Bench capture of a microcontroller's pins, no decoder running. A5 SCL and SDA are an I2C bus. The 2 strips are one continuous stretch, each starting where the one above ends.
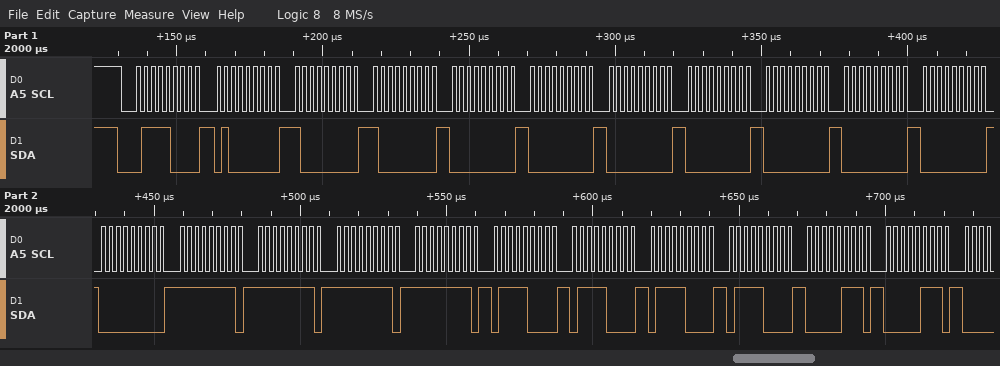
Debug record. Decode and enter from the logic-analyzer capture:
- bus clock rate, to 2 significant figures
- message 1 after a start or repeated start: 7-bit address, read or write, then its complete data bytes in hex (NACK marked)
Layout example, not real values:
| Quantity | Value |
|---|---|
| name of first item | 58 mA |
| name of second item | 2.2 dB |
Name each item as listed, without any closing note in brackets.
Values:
| Quantity | Value |
|---|---|
| bus clock rate, to 2 significant figures | 400 kHz |
| message 1 after a start or repeated start: 7-bit address, read or write, then its complete data bytes in hex | 0x3C write: 40 80 80 00 00 00 00 00 00 00 00 FF FF FF FF 78 78 78 78 07 07 |
